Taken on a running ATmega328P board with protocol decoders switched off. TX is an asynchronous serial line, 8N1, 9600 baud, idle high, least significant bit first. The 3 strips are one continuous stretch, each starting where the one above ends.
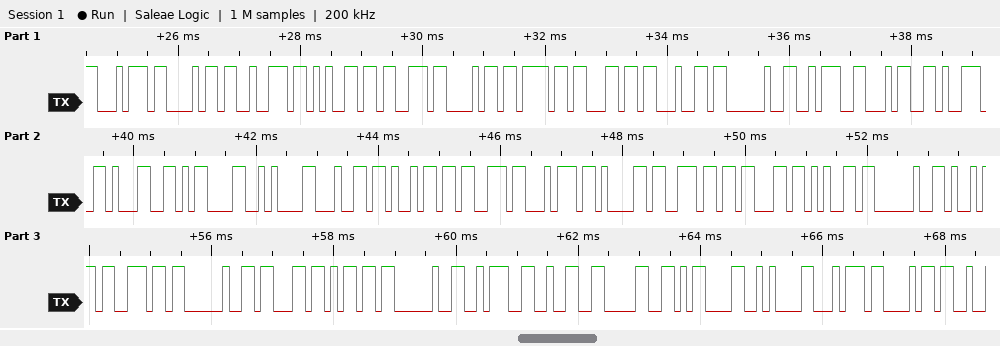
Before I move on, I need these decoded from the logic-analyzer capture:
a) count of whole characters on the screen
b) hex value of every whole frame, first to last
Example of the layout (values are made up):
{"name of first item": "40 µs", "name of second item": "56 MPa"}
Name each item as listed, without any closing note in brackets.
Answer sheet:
{"count of whole characters on the screen": "38", "hex value of every whole frame, first to last": "74 68 72 65 73 68 6F 6C 64 20 3A 34 39 31 0D 0A 64 69 73 74 61 6E 63 65 20 69 6E 20 63 6D 20 3A 32 30 0D 0A 74 68"}
